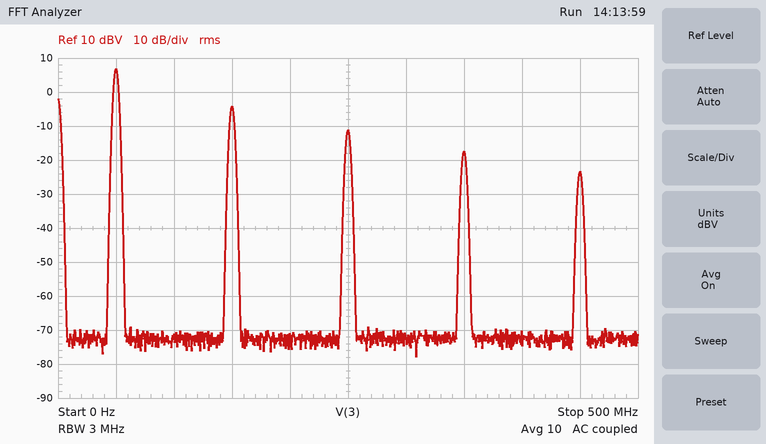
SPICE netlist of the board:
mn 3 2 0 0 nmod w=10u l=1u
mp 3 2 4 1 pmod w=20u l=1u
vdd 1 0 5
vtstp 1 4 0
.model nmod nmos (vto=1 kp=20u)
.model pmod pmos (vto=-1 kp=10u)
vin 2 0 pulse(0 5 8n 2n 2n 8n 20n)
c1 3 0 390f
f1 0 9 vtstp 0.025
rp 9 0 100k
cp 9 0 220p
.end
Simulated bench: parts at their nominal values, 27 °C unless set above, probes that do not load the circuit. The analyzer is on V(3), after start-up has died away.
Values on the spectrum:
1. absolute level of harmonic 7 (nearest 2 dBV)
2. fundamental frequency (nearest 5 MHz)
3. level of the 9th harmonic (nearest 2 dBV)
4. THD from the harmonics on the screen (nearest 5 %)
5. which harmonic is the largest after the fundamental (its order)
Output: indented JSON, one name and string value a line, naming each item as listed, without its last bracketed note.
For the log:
{
  "absolute level of harmonic 7": "-18 dBV",
  "fundamental frequency": "50 MHz",
  "level of the 9th harmonic": "-24 dBV",
  "THD from the harmonics on the screen": "30 %",
  "which harmonic is the largest after the fundamental": "3"
}
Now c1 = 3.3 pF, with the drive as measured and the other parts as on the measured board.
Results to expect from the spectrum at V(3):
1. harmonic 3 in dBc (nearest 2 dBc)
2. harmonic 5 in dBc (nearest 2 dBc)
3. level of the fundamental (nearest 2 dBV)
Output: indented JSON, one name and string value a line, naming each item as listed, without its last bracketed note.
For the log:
{
  "harmonic 3 in dBc": "-22 dBc",
  "harmonic 5 in dBc": "-32 dBc",
  "level of the fundamental": "0 dBV"
}
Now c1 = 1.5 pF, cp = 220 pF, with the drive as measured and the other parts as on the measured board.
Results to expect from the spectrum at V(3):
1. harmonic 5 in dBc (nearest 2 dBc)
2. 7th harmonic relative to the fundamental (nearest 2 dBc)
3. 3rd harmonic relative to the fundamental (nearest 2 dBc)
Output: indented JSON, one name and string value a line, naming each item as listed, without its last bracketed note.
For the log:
{
  "harmonic 5 in dBc": "-30 dBc",
  "7th harmonic relative to the fundamental": "-38 dBc",
  "3rd harmonic relative to the fundamental": "-18 dBc"
}
